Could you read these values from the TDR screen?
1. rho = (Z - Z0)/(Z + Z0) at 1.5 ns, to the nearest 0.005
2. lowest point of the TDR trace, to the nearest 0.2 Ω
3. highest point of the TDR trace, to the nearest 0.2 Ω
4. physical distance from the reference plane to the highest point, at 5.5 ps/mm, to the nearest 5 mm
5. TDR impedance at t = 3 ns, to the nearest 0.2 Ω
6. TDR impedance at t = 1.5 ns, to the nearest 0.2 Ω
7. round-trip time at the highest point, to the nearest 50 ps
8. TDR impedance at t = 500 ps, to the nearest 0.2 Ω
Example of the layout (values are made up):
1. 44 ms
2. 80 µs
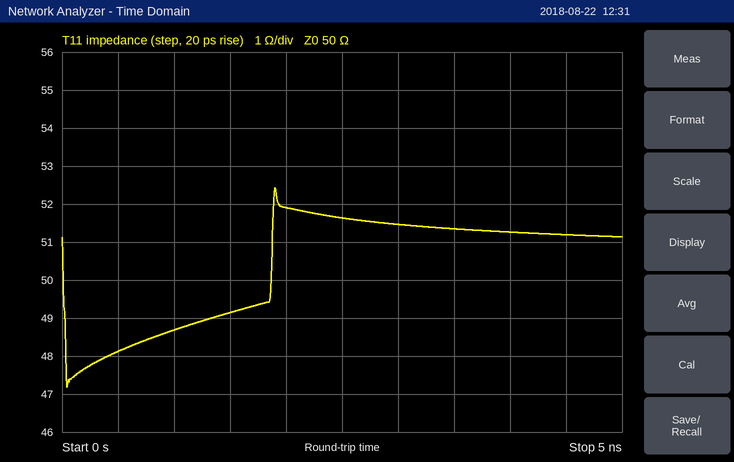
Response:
1. -0.010
2. 47.2 Ω
3. 52.4 Ω
4. 175 mm
5. 51.4 Ω
6. 49.2 Ω
7. 1.90 ns
8. 48.2 Ω
